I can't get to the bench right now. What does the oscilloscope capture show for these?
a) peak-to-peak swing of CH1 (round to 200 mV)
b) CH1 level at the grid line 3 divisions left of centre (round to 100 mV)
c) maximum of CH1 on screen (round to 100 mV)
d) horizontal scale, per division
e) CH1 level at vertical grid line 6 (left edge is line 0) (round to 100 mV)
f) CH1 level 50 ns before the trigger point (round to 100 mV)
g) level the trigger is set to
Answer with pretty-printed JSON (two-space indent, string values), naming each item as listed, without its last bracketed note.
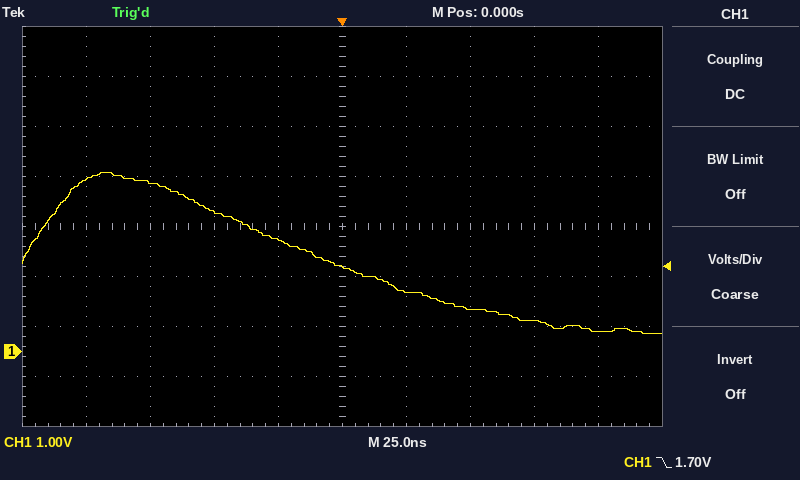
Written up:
{
  "peak-to-peak swing of CH1": "3.2 V",
  "CH1 level at the grid line 3 divisions left of centre": "3.4 V",
  "maximum of CH1 on screen": "3.6 V",
  "horizontal scale, per division": "25 ns",
  "CH1 level at vertical grid line 6 (left edge is line 0)": "1.2 V",
  "CH1 level 50 ns before the trigger point": "2.8 V",
  "level the trigger is set to": "1.70 V"
}
